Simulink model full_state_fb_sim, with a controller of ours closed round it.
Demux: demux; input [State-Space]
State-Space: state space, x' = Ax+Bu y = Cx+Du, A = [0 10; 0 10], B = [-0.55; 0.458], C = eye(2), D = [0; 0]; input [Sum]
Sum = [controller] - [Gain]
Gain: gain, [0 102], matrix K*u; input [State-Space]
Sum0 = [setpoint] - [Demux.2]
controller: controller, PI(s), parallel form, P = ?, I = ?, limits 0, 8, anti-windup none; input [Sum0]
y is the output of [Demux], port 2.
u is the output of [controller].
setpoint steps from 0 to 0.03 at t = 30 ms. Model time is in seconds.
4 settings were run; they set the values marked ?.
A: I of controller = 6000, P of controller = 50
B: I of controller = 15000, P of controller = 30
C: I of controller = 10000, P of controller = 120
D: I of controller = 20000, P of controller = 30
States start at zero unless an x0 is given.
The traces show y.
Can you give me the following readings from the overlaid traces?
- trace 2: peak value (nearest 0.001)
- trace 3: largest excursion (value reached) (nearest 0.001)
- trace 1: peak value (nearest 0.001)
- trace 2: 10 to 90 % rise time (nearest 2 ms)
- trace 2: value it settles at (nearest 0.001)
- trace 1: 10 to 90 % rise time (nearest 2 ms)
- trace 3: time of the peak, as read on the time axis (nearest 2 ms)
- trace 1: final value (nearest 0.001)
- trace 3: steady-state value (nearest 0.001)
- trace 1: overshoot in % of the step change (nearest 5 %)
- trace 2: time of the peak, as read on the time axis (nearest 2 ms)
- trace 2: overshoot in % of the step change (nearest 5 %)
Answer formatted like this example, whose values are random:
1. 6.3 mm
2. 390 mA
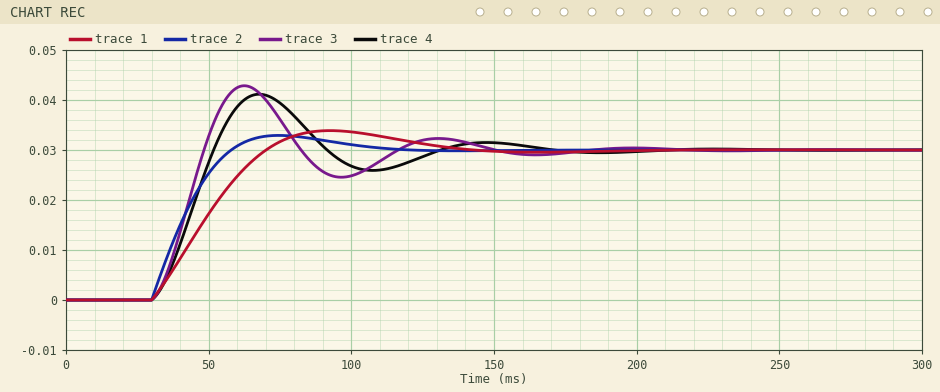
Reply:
1. 0.033
2. 0.043
3. 0.034
4. 20 ms
5. 0.030
6. 30 ms
7. 62 ms
8. 0.030
9. 0.030
10. 15 %
11. 74 ms
12. 10 %
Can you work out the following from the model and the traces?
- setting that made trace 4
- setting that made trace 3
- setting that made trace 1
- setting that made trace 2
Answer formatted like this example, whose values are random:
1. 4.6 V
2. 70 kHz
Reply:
1. B
2. D
3. A
4. C
